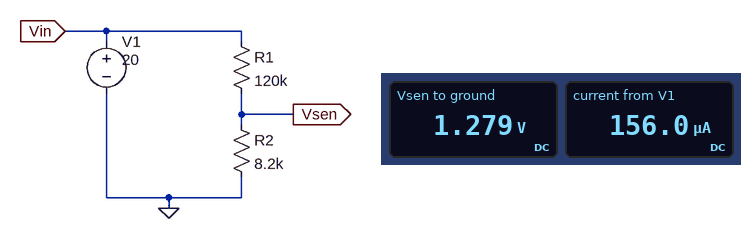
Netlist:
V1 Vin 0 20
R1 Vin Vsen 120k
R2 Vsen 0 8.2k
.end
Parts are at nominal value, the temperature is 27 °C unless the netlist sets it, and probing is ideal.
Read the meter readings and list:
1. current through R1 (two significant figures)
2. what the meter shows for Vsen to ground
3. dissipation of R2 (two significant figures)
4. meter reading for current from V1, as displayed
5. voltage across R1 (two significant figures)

160 µA
1.279 V
200 µW
156.0 µA
19 V
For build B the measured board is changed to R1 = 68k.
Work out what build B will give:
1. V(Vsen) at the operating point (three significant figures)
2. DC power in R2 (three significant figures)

2.15 V
565 µW
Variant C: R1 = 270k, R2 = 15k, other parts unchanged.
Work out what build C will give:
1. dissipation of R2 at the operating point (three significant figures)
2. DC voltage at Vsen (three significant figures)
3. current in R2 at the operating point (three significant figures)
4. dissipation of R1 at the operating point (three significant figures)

73.9 µW
1.05 V
70.2 µA
1.33 mW
